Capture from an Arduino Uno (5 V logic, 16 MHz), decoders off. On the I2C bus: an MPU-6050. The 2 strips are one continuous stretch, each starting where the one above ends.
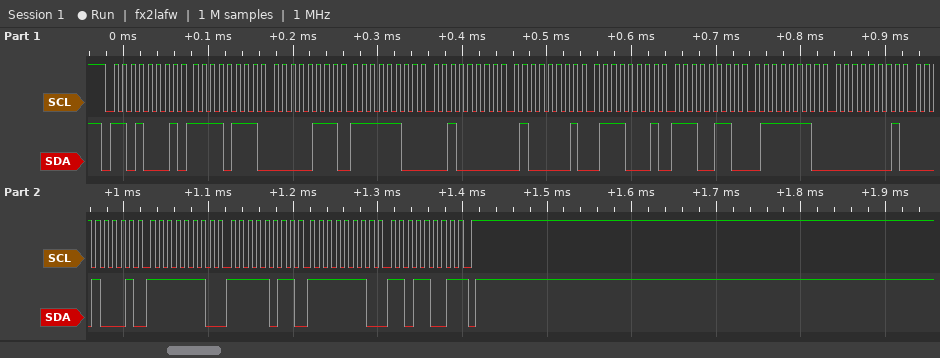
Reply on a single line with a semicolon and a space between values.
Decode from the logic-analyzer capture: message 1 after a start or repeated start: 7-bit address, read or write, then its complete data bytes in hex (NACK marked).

0x68 read: F7 07 FC 20 41 71 E6 7E 01 11 FE FB FE D9 NACK
